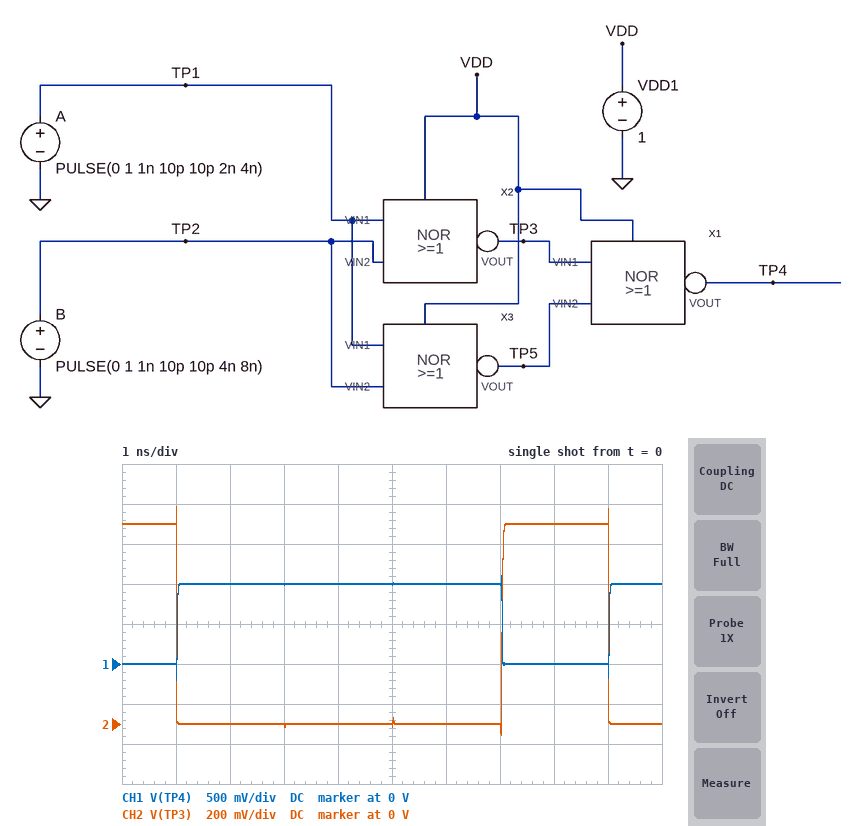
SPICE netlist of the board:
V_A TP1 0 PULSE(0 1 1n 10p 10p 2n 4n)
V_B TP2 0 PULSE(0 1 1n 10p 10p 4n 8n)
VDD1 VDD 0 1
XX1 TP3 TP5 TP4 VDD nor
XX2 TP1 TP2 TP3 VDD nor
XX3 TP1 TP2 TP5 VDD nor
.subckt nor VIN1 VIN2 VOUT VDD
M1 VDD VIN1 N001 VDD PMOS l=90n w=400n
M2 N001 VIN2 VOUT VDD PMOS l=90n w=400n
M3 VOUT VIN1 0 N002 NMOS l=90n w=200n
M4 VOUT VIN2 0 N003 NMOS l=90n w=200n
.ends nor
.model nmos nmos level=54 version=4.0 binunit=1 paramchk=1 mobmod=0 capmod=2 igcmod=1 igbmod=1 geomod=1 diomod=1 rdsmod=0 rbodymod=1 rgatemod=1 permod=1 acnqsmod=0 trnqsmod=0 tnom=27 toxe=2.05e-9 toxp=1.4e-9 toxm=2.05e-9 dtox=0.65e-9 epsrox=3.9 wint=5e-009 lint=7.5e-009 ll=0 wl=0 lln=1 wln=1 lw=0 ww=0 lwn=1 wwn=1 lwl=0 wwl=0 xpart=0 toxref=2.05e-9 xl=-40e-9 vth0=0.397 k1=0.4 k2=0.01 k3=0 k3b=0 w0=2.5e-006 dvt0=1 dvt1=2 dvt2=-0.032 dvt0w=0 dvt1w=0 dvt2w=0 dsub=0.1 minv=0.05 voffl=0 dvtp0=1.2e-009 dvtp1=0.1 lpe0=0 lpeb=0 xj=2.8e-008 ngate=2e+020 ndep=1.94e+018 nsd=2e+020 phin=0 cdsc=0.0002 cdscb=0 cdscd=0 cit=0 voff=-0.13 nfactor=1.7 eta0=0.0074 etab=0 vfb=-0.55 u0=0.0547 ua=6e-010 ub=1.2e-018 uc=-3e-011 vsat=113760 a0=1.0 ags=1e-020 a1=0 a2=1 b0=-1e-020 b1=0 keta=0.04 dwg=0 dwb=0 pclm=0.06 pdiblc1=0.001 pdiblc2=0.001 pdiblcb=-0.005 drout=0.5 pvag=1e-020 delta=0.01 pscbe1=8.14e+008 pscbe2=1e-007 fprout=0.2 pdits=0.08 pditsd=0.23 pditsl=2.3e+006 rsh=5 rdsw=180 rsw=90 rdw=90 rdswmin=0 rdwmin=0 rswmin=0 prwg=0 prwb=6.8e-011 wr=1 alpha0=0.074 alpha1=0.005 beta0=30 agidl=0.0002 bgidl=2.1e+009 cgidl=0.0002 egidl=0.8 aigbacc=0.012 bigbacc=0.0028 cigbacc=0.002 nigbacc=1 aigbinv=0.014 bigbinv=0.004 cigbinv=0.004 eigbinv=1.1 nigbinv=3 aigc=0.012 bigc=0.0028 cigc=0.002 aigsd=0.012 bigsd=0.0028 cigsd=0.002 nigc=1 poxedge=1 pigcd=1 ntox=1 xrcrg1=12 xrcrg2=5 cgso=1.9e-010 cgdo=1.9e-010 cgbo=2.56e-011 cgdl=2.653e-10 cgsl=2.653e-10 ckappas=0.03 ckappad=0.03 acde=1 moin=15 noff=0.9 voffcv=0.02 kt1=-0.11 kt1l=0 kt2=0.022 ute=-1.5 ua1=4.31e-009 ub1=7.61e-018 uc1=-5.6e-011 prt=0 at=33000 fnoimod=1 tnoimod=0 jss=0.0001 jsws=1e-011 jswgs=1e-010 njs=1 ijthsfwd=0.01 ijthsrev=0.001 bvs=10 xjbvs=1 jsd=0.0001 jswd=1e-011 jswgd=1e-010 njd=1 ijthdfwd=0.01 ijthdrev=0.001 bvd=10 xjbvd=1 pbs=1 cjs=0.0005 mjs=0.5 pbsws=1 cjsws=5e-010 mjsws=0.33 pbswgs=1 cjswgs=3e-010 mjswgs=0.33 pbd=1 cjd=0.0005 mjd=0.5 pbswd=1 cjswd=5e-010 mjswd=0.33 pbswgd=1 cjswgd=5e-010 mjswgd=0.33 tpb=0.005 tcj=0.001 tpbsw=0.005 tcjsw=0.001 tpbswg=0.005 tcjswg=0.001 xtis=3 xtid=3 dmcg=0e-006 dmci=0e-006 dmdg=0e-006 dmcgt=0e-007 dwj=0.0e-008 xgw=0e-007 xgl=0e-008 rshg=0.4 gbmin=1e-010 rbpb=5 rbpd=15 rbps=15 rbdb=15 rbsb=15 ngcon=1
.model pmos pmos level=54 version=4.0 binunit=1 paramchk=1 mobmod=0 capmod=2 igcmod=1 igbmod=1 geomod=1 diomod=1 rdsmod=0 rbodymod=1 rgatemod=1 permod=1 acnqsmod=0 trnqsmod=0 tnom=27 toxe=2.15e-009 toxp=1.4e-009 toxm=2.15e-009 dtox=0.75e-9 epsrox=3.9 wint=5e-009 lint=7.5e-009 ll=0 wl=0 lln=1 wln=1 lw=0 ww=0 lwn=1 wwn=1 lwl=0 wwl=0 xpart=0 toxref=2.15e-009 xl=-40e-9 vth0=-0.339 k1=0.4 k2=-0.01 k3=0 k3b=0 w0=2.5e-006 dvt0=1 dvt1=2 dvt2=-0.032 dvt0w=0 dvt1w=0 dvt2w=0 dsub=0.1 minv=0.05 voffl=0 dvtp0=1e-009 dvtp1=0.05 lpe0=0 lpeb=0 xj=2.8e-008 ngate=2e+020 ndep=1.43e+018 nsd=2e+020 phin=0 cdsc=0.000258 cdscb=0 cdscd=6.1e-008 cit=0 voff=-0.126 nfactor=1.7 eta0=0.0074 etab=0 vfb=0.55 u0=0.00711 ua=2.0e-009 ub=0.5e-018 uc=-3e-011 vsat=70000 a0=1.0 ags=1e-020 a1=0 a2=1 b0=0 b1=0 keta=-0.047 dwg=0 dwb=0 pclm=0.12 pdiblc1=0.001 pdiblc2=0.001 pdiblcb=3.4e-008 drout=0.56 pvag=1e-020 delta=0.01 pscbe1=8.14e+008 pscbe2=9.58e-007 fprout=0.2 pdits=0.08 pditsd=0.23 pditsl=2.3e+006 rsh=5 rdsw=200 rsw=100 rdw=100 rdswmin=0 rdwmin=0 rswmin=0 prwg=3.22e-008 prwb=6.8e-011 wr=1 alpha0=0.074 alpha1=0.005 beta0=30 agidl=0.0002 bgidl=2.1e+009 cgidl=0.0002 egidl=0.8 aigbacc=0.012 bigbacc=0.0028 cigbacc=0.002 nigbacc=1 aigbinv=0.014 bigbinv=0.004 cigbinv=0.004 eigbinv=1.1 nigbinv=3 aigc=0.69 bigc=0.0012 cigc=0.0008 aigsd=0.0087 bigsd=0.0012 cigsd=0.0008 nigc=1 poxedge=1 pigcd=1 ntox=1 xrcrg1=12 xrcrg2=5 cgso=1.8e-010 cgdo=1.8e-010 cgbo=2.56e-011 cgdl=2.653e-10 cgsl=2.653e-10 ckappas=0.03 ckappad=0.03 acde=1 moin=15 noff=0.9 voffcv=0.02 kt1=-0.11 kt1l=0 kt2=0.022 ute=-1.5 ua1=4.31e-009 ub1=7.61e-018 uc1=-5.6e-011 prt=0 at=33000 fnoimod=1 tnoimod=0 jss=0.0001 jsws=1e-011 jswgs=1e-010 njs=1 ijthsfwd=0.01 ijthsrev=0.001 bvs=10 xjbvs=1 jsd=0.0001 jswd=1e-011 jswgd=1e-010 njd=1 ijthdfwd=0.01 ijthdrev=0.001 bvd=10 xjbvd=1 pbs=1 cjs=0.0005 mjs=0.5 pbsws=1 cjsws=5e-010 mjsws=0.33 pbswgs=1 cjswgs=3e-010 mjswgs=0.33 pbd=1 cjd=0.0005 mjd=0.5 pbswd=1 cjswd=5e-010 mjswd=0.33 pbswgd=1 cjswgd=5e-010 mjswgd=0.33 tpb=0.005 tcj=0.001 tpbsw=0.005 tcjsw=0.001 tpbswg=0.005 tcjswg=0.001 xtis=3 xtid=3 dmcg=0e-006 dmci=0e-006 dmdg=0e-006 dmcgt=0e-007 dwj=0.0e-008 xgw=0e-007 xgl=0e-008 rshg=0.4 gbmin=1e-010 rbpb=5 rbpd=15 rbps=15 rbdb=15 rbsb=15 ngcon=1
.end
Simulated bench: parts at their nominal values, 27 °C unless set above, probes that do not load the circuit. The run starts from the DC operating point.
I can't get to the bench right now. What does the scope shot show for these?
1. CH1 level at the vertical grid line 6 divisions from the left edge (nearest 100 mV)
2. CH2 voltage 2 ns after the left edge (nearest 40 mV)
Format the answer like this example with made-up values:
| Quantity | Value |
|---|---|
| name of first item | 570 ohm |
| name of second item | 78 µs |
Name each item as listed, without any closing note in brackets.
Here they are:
| Quantity | Value |
|---|---|
| CH1 level at the vertical grid line 6 divisions from the left edge | 1.0 V |
| CH2 voltage 2 ns after the left edge | 0 V |
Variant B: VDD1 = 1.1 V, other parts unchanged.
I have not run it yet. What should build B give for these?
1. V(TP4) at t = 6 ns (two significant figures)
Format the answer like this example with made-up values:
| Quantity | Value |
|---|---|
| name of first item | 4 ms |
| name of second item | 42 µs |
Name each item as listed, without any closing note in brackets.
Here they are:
| Quantity | Value |
|---|---|
| V(TP4) at t = 6 ns | 1.1 V |
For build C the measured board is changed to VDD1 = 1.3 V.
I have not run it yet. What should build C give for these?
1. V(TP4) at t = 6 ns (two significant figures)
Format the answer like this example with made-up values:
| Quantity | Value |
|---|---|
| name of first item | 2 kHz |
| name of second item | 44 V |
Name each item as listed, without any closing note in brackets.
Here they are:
| Quantity | Value |
|---|---|
| V(TP4) at t = 6 ns | 1.3 V |
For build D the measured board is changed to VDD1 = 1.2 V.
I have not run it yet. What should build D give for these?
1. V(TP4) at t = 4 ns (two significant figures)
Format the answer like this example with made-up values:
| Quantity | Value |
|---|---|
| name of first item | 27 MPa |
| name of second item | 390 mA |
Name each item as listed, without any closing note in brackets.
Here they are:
| Quantity | Value |
|---|---|
| V(TP4) at t = 4 ns | 1.2 V |
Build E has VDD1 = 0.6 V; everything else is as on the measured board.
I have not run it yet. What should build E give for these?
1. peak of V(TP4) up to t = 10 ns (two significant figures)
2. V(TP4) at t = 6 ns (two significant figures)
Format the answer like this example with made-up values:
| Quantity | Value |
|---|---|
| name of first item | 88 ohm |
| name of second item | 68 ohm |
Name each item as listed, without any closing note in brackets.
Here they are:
| Quantity | Value |
|---|---|
| peak of V(TP4) up to t = 10 ns | 680 mV |
| V(TP4) at t = 6 ns | 600 mV |
